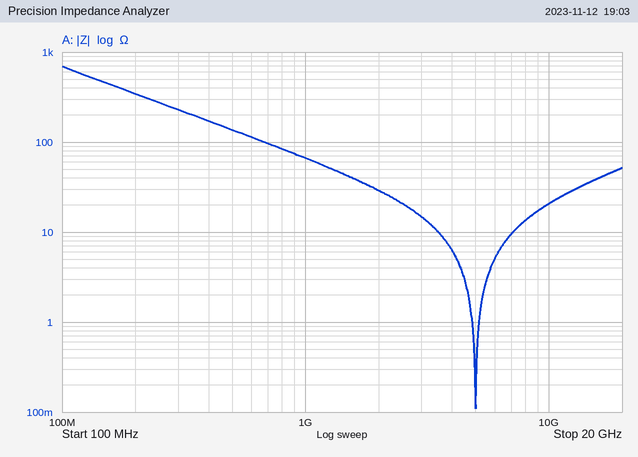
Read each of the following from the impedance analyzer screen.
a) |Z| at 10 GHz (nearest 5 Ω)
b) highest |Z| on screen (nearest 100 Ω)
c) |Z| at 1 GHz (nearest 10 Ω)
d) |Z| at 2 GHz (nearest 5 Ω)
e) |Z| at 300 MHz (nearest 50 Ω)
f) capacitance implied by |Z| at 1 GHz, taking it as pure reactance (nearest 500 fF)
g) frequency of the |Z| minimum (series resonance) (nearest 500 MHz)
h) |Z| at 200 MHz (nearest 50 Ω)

20 Ω
700 Ω
70 Ω
30 Ω
250 Ω
2.5 pF
5.0 GHz
350 Ω
